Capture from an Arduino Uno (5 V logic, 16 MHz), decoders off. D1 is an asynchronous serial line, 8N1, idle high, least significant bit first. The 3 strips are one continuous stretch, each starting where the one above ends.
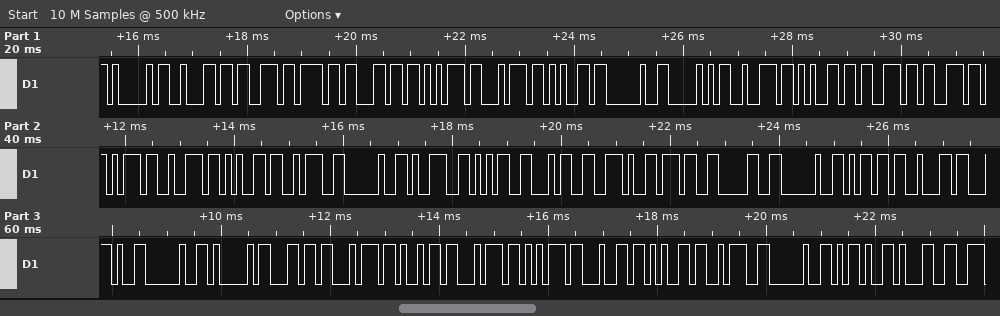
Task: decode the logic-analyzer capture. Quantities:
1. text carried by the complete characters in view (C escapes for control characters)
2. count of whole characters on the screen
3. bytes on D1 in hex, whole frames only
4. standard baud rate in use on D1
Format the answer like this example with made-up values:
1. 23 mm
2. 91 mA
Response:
1. "Absolute Pressure: 954.70 mb, Altitude: -1"
2. 42
3. 41 62 73 6F 6C 75 74 65 20 50 72 65 73 73 75 72 65 3A 20 39 35 34 2E 37 30 20 6D 62 2C 20 41 6C 74 69 74 75 64 65 3A 20 2D 31
4. 9600 baud
